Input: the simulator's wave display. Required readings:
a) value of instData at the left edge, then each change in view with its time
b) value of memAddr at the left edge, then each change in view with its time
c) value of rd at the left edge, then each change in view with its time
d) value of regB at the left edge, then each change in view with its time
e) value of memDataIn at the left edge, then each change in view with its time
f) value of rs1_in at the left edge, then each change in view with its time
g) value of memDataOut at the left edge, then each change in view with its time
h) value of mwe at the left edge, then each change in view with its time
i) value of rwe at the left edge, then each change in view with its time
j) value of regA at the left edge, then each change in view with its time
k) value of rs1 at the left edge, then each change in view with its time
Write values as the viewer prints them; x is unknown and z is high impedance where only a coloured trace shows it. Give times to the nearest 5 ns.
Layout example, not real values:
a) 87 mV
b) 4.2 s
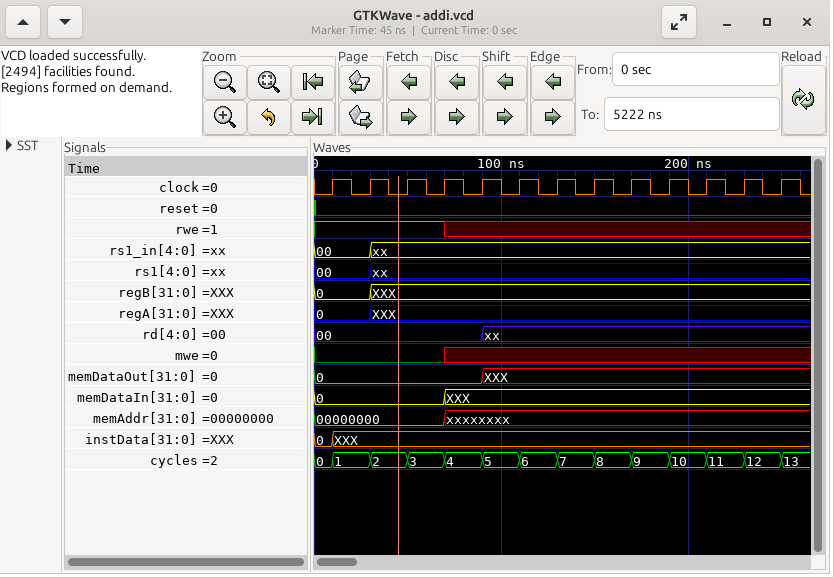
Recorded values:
a) 0, XXX at 10 ns
b) 00000000, xxxxxxxx at 70 ns
c) 00, xx at 90 ns
d) 0, XXX at 30 ns
e) 0, XXX at 70 ns
f) 00, xx at 30 ns
g) 0, XXX at 90 ns
h) 0, x at 70 ns
i) 1, x at 70 ns
j) 0, XXX at 30 ns
k) 00, xx at 30 ns
